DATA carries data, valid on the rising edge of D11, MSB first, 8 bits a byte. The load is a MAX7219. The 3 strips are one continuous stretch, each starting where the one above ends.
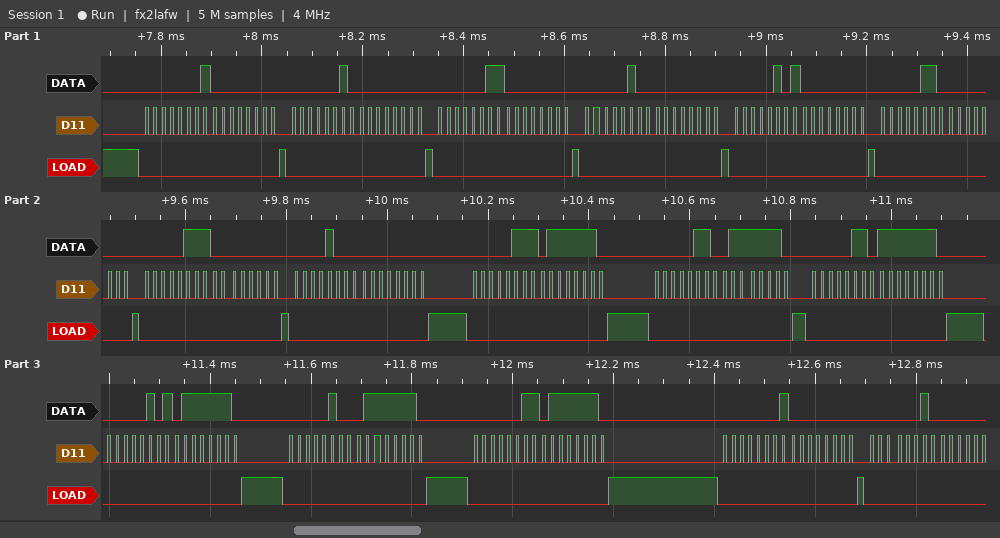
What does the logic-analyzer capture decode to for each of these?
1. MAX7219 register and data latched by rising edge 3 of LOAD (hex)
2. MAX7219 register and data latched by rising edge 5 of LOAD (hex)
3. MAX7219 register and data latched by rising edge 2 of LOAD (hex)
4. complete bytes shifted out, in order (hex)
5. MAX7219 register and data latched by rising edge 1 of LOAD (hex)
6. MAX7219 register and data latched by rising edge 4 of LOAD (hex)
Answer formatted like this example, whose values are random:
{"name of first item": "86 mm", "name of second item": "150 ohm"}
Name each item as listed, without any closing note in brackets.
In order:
{"MAX7219 register and data latched by rising edge 3 of LOAD": "register 0x3, data 0x00", "MAX7219 register and data latched by rising edge 5 of LOAD": "register 0x5, data 0x00", "MAX7219 register and data latched by rising edge 2 of LOAD": "register 0x2, data 0x00", "complete bytes shifted out, in order": "0x01 0x00 0x02 0x00 0x03 0x00 0x04 0x00 0x05 0x00 0x06 0x00 0x07 0x00 0x08 0x00 0x07 0x7E 0x06 0x7E 0x06 0xFE 0x05 0x7E 0x04 0x7E 0x03 0x7E 0x01 0x00 0x02", "MAX7219 register and data latched by rising edge 1 of LOAD": "register 0x1, data 0x00", "MAX7219 register and data latched by rising edge 4 of LOAD": "register 0x4, data 0x00"}
